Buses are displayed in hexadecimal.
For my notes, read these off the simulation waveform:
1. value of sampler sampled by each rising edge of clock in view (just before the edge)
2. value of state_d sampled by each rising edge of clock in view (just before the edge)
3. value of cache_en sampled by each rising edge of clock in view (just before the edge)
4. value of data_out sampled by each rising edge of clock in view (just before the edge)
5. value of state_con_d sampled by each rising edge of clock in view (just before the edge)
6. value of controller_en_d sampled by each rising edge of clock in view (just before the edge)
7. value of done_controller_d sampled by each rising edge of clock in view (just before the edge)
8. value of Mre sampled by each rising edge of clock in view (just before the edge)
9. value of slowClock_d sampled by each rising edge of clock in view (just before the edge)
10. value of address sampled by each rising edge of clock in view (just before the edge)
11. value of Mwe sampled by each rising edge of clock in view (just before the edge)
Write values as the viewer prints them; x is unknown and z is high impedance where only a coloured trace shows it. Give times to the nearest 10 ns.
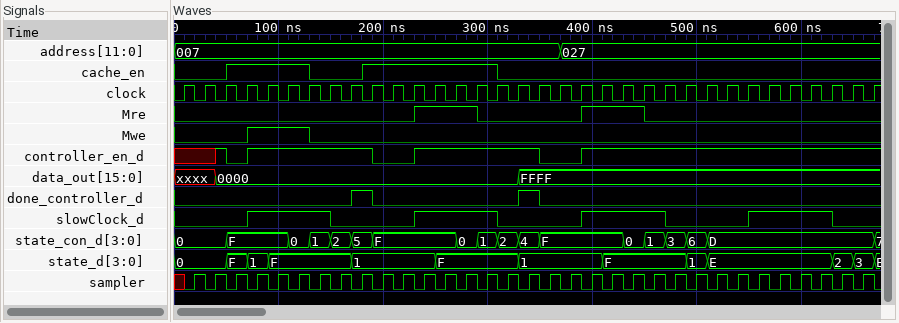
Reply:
x 1 1 1 1 1 1 1 1 1 1 1 1 1 1 1 1 1 1 1 1 1 1 1 1 1 1 1 1 1 1 1 1 1
0, 0, 0, F, 1, F, F, F, F, 1, 1, 1, 1, F, F, F, F, 1, 1, 1, 1, F, F, F, F, 1, E, E, E, E, E, E, 2, 3
0 0 0 1 1 1 1 0 0 1 1 1 1 1 1 1 0 0 0 0 0 0 0 0 0 0 0 0 0 0 0 0 0 0
xxxx, xxxx, 0000, 0000, 0000, 0000, 0000, 0000, 0000, 0000, 0000, 0000, 0000, 0000, 0000, 0000, 0000, FFFF, FFFF, FFFF, FFFF, FFFF, FFFF, FFFF, FFFF, FFFF, FFFF, FFFF, FFFF, FFFF, FFFF, FFFF, FFFF, FFFF
0, 0, 0, F, F, F, 0, 1, 2, 5, F, F, F, F, 0, 1, 2, 4, F, F, F, F, 0, 1, 3, 6, D, D, D, D, D, D, D, D
x x 1 0 1 1 1 1 1 1 0 0 1 1 1 1 1 1 0 0 1 1 1 1 1 1 1 1 1 1 1 1 1 1
0 0 0 0 0 0 0 0 0 1 0 0 0 0 0 0 0 1 0 0 0 0 0 0 0 0 0 0 0 0 0 0 0 0
0 0 0 0 0 0 0 0 0 0 0 0 1 1 1 0 0 0 0 0 1 1 1 0 0 0 0 0 0 0 0 0 0 0
0 0 0 0 1 1 1 1 0 0 0 0 1 1 1 1 0 0 0 0 1 1 1 1 0 0 0 0 1 1 1 1 0 0
007, 007, 007, 007, 007, 007, 007, 007, 007, 007, 007, 007, 007, 007, 007, 007, 007, 007, 007, 027, 027, 027, 027, 027, 027, 027, 027, 027, 027, 027, 027, 027, 027, 027
0 0 0 0 1 1 1 0 0 0 0 0 0 0 0 0 0 0 0 0 0 0 0 0 0 0 0 0 0 0 0 0 0 0
